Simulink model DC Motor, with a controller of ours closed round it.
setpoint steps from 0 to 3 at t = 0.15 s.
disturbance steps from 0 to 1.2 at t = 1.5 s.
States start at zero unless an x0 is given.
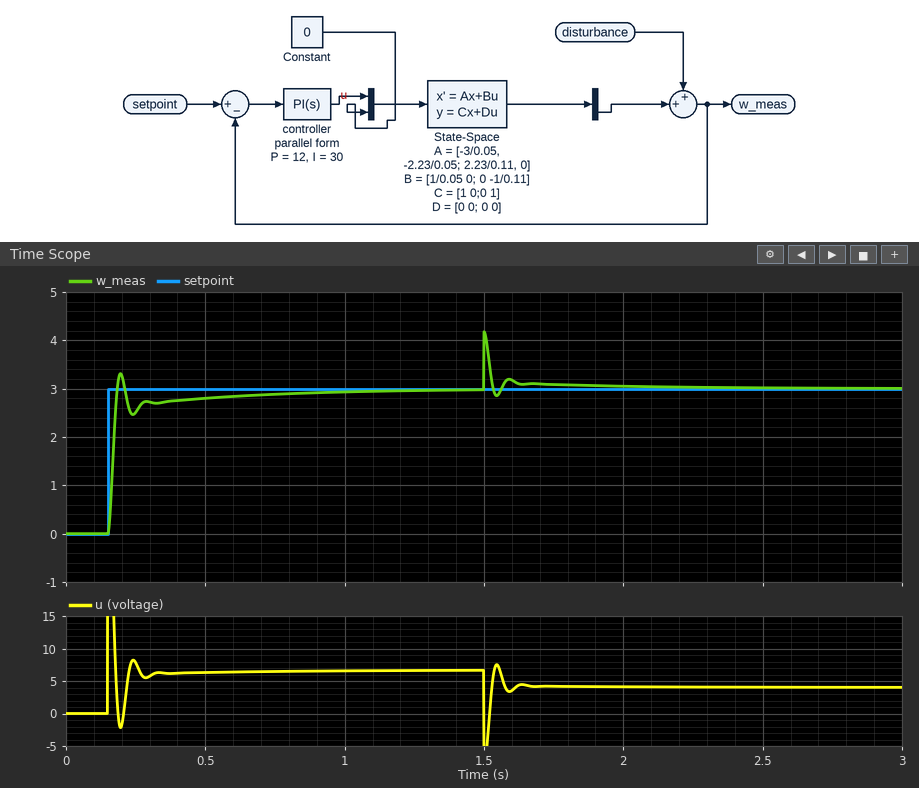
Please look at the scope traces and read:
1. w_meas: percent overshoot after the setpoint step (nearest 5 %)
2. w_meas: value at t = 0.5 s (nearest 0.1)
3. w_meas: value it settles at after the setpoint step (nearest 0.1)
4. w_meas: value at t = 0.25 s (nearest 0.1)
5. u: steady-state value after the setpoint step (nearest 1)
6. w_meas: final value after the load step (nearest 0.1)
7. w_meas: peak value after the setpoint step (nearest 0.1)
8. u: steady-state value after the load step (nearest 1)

10 %
2.8
3.0
2.5
7
3.0
3.3
4
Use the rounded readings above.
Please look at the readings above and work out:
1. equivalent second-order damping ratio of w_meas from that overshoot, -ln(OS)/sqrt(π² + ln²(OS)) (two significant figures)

0.59
